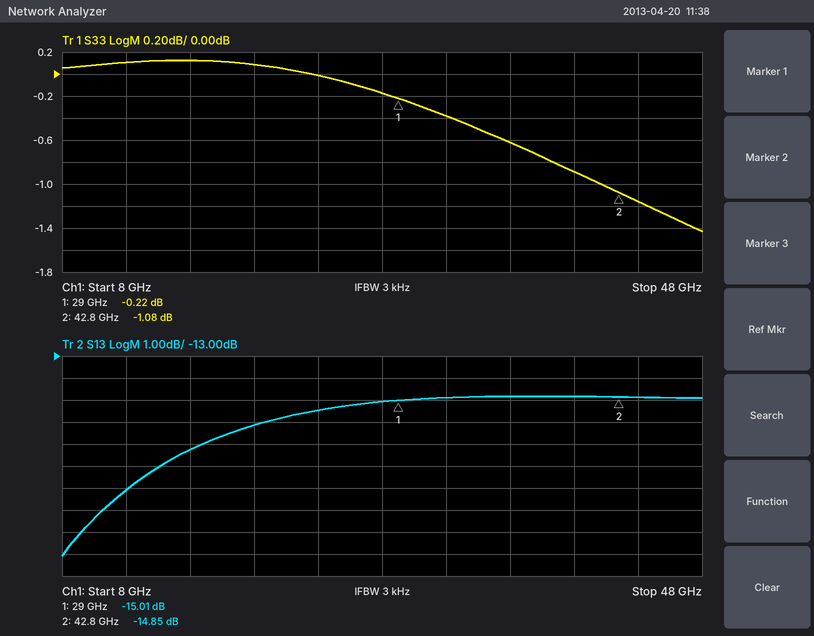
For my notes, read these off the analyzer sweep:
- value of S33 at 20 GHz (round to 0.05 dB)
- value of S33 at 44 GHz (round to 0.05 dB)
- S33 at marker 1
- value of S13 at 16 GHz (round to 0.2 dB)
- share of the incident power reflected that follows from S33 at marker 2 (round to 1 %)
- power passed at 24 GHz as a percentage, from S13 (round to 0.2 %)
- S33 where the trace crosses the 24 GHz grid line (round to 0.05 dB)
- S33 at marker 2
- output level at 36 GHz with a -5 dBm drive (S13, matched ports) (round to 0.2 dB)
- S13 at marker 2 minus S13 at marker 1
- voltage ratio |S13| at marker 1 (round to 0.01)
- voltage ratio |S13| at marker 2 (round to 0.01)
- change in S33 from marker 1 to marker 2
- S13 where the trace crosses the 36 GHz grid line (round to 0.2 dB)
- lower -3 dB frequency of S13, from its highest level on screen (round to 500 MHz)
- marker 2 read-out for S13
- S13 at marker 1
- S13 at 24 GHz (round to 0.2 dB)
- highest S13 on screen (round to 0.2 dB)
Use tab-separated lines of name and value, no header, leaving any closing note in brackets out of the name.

value of S33 at 20 GHz	0.10 dB
value of S33 at 44 GHz	-1.15 dB
S33 at marker 1	-0.22 dB
value of S13 at 16 GHz	-17.2 dB
share of the incident power reflected that follows from S33 at marker 2	78 %
power passed at 24 GHz as a percentage, from S13	2.8 %
S33 where the trace crosses the 24 GHz grid line	0.00 dB
S33 at marker 2	-1.08 dB
output level at 36 GHz with a -5 dBm drive (S13, matched ports)	-19.8 dBm
S13 at marker 2 minus S13 at marker 1	0.16 dB
voltage ratio |S13| at marker 1	0.18
voltage ratio |S13| at marker 2	0.18
change in S33 from marker 1 to marker 2	-0.86 dB
S13 where the trace crosses the 36 GHz grid line	-14.8 dB
lower -3 dB frequency of S13, from its highest level on screen	14.5 GHz
marker 2 read-out for S13	-14.85 dB
S13 at marker 1	-15.01 dB
S13 at 24 GHz	-15.4 dB
highest S13 on screen	-14.8 dB
